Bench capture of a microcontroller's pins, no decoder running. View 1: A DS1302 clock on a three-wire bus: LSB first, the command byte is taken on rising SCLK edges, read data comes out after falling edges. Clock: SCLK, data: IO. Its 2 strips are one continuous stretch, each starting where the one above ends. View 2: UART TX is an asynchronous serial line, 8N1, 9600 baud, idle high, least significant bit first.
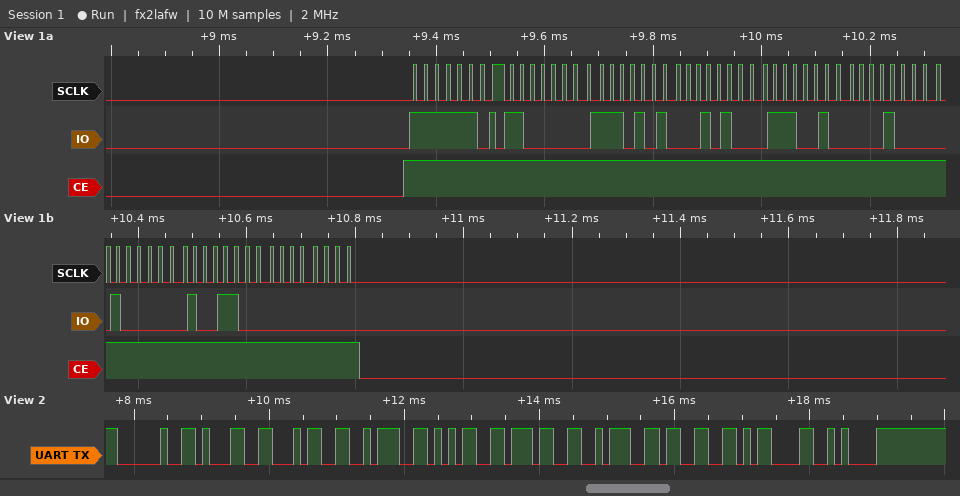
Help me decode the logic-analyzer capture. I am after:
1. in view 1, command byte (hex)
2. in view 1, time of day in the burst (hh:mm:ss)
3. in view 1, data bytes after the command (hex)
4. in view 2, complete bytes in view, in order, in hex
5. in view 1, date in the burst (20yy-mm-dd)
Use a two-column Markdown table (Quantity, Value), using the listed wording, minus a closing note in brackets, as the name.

| Quantity | Value |
|---|---|
| in view 1, command byte | 0xBF |
| in view 1, time of day in the burst | 14:57:03 |
| in view 1, data bytes after the command | 03 57 14 27 08 02 19 00 |
| in view 2, complete bytes in view, in order, in hex | 0x20 0x31 0x34 0x3A 0x35 0x37 0x3A 0x33 0x0D 0x0A |
| in view 1, date in the burst | 2019-08-27 |
